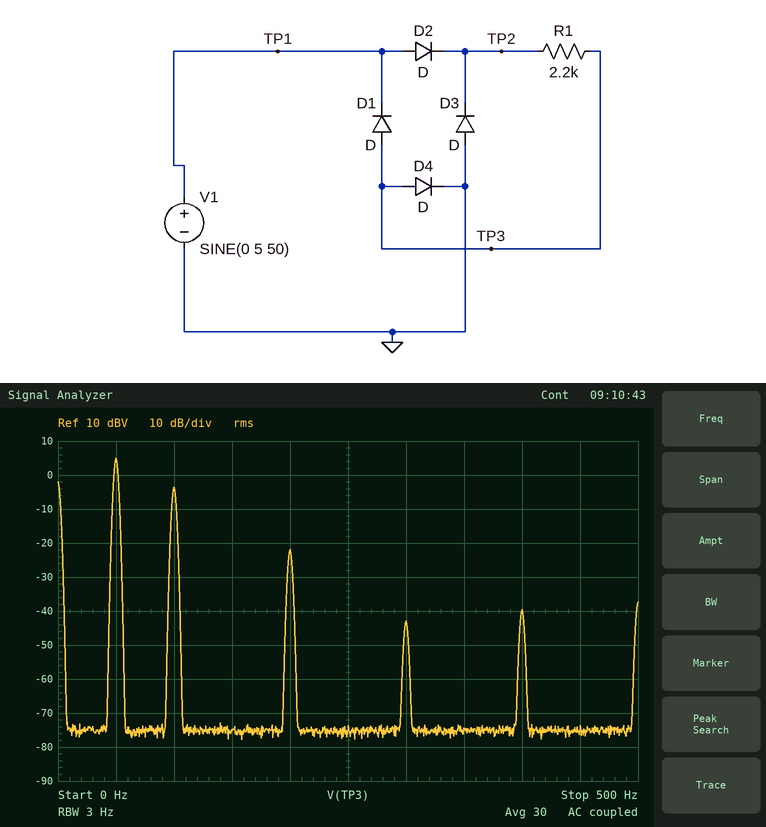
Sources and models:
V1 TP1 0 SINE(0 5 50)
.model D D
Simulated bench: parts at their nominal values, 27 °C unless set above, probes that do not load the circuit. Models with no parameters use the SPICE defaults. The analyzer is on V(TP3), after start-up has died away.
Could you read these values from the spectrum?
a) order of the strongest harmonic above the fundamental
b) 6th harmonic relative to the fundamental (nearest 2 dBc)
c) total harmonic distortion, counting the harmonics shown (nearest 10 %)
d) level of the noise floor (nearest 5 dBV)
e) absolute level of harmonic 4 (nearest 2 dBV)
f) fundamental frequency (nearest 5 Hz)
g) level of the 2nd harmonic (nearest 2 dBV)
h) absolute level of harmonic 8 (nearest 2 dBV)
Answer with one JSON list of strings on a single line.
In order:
["2", "-48 dBc", "40 %", "-75 dBV", "-22 dBV", "50 Hz", "-4 dBV", "-40 dBV"]
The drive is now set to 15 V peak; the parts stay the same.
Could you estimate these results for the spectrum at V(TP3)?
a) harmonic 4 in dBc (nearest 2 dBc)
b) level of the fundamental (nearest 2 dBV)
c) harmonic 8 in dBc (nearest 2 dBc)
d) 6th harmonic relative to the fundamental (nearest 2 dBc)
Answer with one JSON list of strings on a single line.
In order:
["-22 dBc", "14 dBV", "-36 dBc", "-30 dBc"]
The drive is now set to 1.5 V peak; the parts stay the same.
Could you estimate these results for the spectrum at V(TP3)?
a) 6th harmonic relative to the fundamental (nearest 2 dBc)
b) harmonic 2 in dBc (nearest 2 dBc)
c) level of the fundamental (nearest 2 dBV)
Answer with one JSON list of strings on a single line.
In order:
["-50 dBc", "-20 dBc", "-6 dBV"]
